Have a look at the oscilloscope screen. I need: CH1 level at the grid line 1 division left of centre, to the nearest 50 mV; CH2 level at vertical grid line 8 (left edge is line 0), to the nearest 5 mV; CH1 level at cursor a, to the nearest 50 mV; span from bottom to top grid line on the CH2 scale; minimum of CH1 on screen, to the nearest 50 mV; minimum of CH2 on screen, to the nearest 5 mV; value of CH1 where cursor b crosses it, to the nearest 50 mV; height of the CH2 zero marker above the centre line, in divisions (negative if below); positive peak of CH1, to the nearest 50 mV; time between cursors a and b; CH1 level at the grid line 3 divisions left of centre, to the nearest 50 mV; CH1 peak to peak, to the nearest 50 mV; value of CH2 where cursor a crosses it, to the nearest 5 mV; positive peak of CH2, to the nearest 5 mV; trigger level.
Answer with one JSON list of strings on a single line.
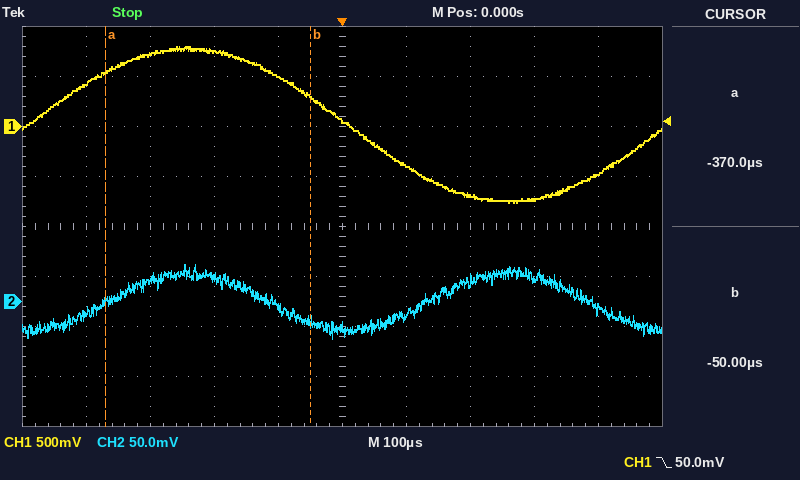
["500 mV", "25 mV", "550 mV", "400 mV", "-750 mV", "-35 mV", "300 mV", "-1.5 div", "800 mV", "320 µs", "700 mV", "1.55 V", "0 mV", "35 mV", "50.0 mV"]
